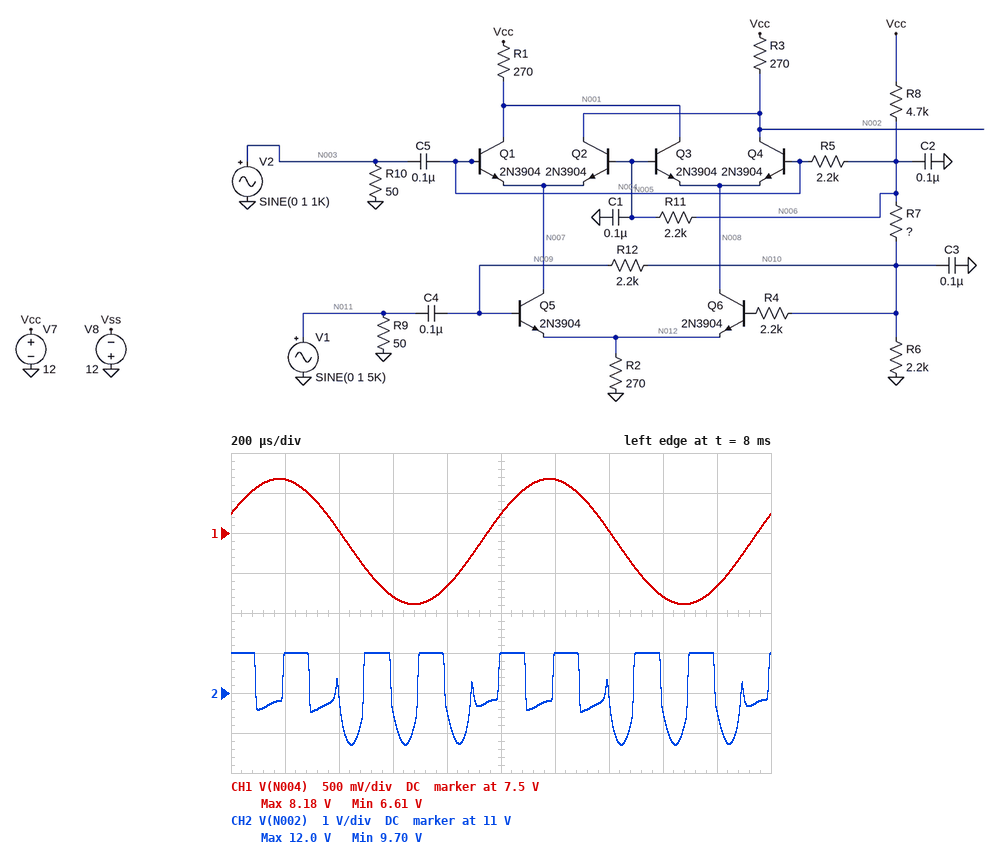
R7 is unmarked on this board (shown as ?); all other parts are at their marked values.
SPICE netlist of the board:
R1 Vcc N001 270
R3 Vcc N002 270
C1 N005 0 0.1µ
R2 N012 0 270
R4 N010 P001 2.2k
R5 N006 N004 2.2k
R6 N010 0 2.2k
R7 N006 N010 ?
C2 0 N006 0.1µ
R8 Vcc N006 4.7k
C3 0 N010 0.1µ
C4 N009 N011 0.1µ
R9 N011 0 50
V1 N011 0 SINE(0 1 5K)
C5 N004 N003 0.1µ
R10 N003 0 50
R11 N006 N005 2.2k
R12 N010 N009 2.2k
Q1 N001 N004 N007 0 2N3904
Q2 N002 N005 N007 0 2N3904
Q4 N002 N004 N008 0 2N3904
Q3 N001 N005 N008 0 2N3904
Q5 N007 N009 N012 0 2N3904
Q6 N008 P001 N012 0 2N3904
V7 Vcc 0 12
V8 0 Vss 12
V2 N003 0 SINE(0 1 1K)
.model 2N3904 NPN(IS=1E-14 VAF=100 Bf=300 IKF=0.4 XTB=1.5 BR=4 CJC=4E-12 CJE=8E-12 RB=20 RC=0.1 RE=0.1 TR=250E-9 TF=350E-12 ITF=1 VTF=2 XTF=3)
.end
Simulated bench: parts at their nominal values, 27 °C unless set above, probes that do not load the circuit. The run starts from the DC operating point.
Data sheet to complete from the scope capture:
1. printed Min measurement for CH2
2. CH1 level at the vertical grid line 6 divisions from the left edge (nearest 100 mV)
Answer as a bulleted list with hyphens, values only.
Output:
- 9.70 V
- 8.2 V
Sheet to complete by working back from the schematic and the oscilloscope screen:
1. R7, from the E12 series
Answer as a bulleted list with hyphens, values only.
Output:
- 5.6 kΩ
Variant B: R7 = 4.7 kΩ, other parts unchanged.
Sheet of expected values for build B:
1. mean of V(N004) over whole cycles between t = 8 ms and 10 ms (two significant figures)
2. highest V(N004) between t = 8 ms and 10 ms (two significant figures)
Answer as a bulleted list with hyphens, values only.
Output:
- 7.0 V
- 7.8 V
